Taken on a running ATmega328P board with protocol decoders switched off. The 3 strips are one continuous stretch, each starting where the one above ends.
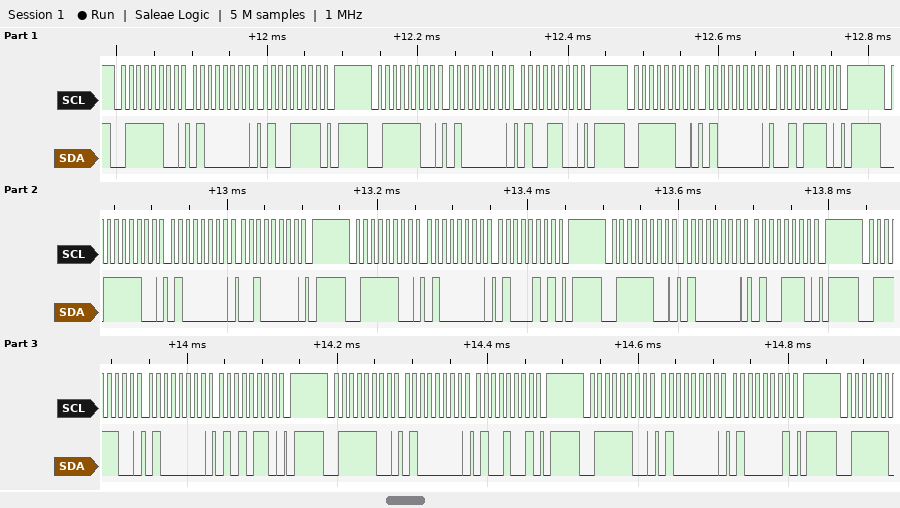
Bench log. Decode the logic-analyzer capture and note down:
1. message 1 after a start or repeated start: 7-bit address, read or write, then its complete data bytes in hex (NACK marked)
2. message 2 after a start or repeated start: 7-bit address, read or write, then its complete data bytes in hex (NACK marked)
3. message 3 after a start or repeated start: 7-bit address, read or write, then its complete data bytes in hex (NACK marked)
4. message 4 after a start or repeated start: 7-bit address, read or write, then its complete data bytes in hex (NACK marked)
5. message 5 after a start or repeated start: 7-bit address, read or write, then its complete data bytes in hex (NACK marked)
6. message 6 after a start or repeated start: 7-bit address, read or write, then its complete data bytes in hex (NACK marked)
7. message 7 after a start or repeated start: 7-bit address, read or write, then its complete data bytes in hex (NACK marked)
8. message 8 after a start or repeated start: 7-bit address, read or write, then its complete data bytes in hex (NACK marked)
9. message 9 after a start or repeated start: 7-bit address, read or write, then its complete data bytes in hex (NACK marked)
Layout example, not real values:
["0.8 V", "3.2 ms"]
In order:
["0x3E write: 40 4F", "0x3E write: 40 4C", "0x3E write: 40 2E", "0x3E write: 40 20", "0x3E write: 40 45", "0x3E write: 40 4E", "0x3E write: 40 56", "0x3E write: 40 49", "0x3E write: 40 41"]
